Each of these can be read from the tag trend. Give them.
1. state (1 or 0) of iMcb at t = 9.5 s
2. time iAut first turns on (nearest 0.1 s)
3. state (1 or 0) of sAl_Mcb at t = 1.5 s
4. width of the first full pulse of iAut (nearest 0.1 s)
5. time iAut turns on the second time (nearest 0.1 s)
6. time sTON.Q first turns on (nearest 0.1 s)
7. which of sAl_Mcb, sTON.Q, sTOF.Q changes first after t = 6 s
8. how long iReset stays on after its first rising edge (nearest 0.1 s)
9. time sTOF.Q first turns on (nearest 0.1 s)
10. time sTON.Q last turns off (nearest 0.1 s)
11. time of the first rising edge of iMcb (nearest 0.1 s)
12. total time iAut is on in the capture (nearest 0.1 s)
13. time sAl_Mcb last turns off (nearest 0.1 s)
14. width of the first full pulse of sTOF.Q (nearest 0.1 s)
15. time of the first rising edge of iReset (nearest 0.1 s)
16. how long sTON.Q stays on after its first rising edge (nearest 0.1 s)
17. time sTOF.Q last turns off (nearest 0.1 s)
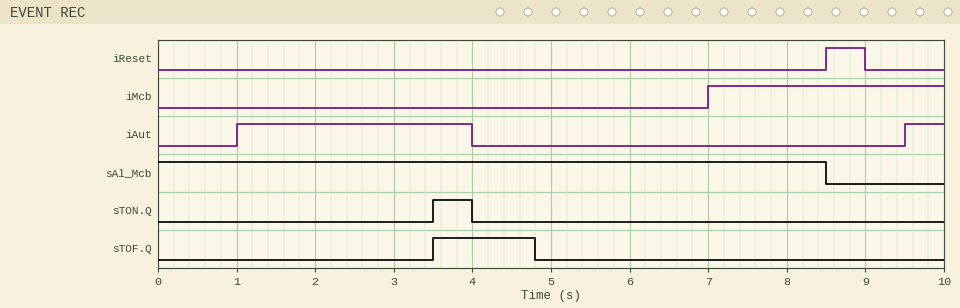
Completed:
1
1.0 s
1
3.0 s
9.5 s
3.5 s
sAl_Mcb
0.5 s
3.5 s
4.0 s
7.0 s
3.5 s
8.5 s
1.3 s
8.5 s
0.5 s
4.8 s
